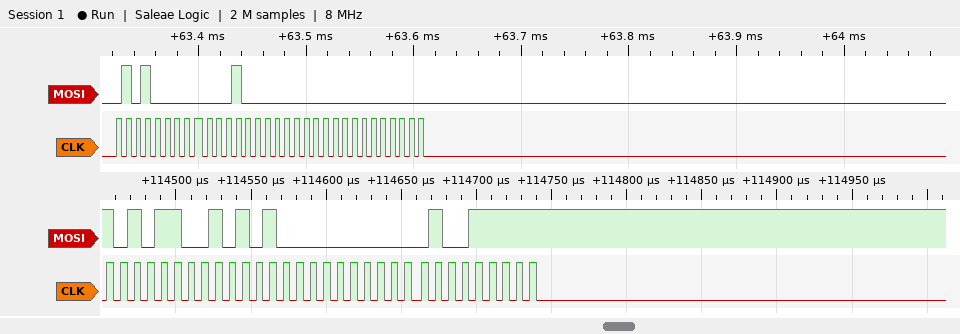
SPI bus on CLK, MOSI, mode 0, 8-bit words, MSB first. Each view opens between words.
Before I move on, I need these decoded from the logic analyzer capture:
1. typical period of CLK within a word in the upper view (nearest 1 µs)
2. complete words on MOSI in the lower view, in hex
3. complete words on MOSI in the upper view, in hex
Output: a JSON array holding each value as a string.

["9 µs", "AC, A8, 00, 9F", "50, 08, 00, 00"]
